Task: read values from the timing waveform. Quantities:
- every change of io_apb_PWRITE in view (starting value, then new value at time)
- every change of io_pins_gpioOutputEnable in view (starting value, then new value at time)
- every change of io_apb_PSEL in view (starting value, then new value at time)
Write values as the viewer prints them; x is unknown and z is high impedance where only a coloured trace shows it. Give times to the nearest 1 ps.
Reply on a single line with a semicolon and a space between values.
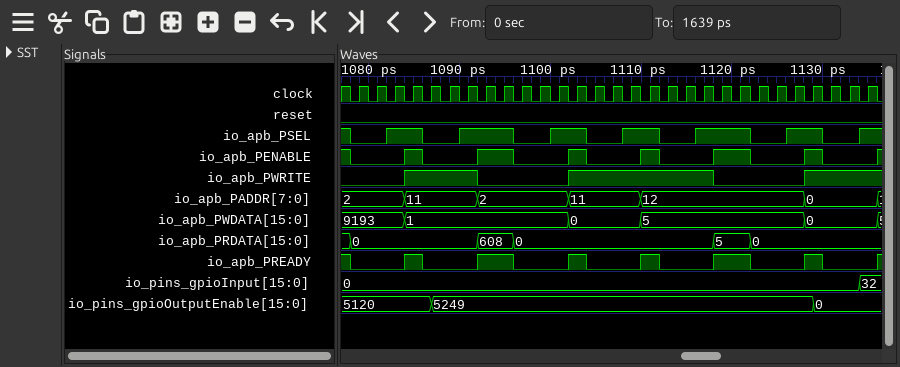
0, 1 at 1084 ps, 0 at 1092 ps, 1 at 1102 ps, 0 at 1118 ps, 1 at 1128 ps; 5120, 5249 at 1087 ps, 0 at 1129 ps; 1, 0 at 1078 ps, 1 at 1082 ps, 0 at 1086 ps, 1 at 1090 ps, 0 at 1096 ps, 1 at 1100 ps, 0 at 1104 ps, 1 at 1108 ps, 0 at 1112 ps, 1 at 1116 ps, 0 at 1122 ps, 1 at 1126 ps, 0 at 1130 ps, 1 at 1134 ps
